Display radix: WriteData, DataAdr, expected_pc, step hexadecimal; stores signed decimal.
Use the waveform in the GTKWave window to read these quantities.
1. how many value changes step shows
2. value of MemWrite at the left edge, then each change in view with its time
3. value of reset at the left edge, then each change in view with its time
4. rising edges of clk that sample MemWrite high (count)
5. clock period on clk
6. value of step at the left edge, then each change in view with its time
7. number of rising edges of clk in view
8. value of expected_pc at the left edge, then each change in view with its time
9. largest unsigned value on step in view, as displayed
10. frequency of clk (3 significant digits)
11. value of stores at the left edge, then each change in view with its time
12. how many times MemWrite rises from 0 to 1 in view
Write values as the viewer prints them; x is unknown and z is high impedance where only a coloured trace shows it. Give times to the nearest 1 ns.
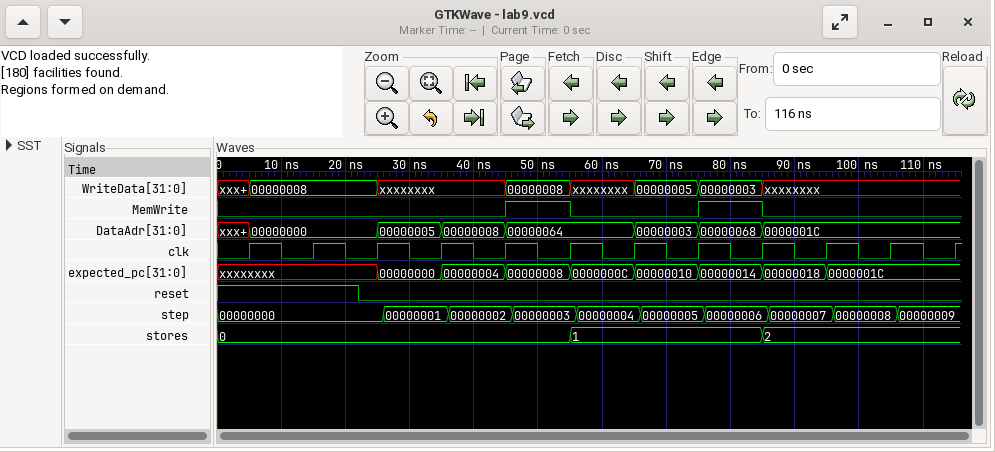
9
0, 1 at 45 ns, 0 at 55 ns, 1 at 75 ns, 0 at 85 ns
1, 0 at 22 ns
2
10 ns
00000000, 00000001 at 26 ns, 00000002 at 36 ns, 00000003 at 46 ns, 00000004 at 56 ns, 00000005 at 66 ns, 00000006 at 76 ns, 00000007 at 86 ns, 00000008 at 96 ns, 00000009 at 106 ns
12
xxxxxxxx, 00000000 at 25 ns, 00000004 at 35 ns, 00000008 at 45 ns, 0000000C at 55 ns, 00000010 at 65 ns, 00000014 at 75 ns, 00000018 at 85 ns, 0000001C at 95 ns
00000009
100 MHz
0, 1 at 55 ns, 2 at 85 ns
2
